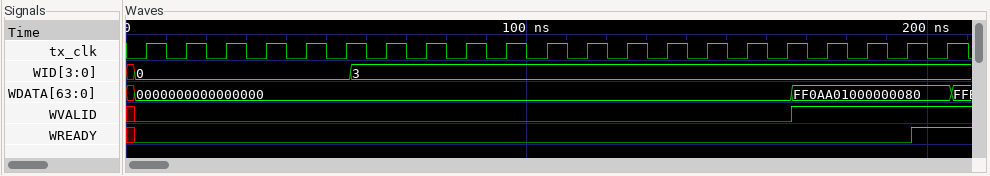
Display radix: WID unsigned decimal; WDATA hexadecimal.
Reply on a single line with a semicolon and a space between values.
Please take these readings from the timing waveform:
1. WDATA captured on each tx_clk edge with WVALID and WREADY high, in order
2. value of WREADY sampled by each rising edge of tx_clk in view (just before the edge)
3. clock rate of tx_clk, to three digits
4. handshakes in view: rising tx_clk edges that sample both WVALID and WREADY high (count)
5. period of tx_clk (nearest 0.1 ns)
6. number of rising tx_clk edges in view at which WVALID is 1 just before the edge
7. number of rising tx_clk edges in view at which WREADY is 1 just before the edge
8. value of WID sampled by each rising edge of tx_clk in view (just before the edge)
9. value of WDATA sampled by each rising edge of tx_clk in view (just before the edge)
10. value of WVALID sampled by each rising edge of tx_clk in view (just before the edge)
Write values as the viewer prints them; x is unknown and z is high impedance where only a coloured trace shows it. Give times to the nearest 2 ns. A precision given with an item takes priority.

FF0AA01000000080; 0 0 0 0 0 0 0 0 0 0 0 0 0 0 0 0 0 0 0 0 1; 100 MHz; 1; 10 ns; 4; 1; 0, 0, 0, 0, 0, 0, 3, 3, 3, 3, 3, 3, 3, 3, 3, 3, 3, 3, 3, 3, 3; 0000000000000000, 0000000000000000, 0000000000000000, 0000000000000000, 0000000000000000, 0000000000000000, 0000000000000000, 0000000000000000, 0000000000000000, 0000000000000000, 0000000000000000, 0000000000000000, 0000000000000000, 0000000000000000, 0000000000000000, 0000000000000000, 0000000000000000, FF0AA01000000080, FF0AA01000000080, FF0AA01000000080, FF0AA01000000080; 0 0 0 0 0 0 0 0 0 0 0 0 0 0 0 0 0 1 1 1 1
